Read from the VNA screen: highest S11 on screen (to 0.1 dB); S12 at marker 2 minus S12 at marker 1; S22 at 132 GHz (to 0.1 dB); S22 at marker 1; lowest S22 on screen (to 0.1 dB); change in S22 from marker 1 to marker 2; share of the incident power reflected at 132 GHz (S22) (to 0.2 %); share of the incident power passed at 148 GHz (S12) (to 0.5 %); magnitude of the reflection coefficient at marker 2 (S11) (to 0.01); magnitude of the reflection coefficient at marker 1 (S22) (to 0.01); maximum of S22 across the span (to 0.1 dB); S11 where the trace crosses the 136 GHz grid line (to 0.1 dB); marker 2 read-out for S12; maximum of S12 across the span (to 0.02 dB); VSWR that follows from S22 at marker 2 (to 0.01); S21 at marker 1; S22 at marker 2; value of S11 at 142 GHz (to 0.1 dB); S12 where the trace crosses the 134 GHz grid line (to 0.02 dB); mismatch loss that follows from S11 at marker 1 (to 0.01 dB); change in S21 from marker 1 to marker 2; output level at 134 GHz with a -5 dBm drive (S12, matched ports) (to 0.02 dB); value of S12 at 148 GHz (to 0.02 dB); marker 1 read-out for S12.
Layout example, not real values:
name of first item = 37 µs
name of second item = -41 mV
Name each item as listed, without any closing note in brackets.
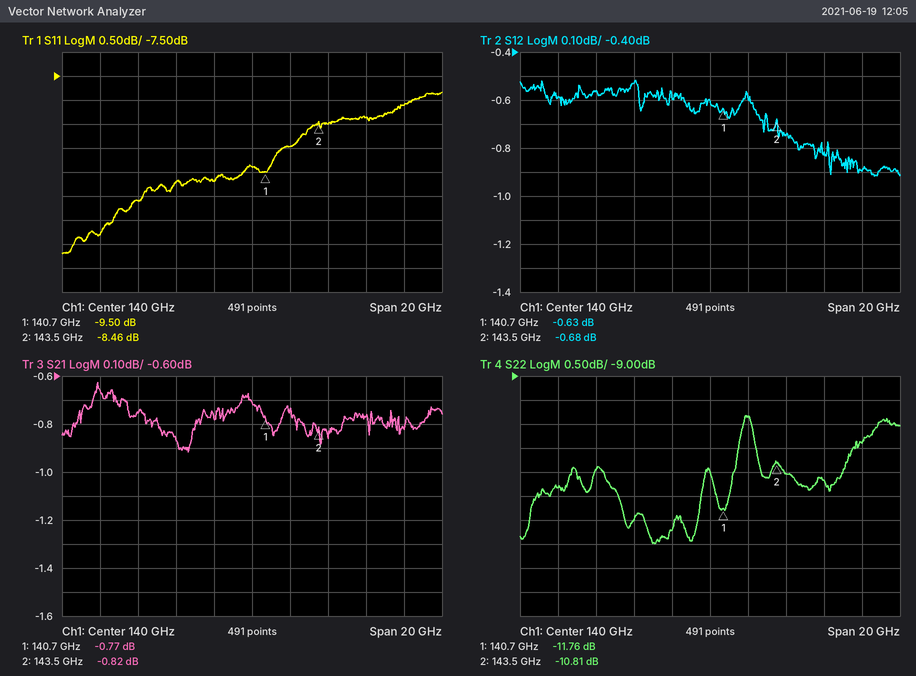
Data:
highest S11 on screen = -7.8 dB
S12 at marker 2 minus S12 at marker 1 = -0.05 dB
S22 at 132 GHz = -11.3 dB
S22 at marker 1 = -11.76 dB
lowest S22 on screen = -12.5 dB
change in S22 from marker 1 to marker 2 = 0.95 dB
share of the incident power reflected at 132 GHz (S22) = 7.4 %
share of the incident power passed at 148 GHz (S12) = 81.5 %
magnitude of the reflection coefficient at marker 2 (S11) = 0.38
magnitude of the reflection coefficient at marker 1 (S22) = 0.26
maximum of S22 across the span = -9.8 dB
S11 where the trace crosses the 136 GHz grid line = -9.7 dB
marker 2 read-out for S12 = -0.68 dB
maximum of S12 across the span = -0.52 dB
VSWR that follows from S22 at marker 2 = 1.81
S21 at marker 1 = -0.77 dB
S22 at marker 2 = -10.81 dB
value of S11 at 142 GHz = -9.0 dB
S12 where the trace crosses the 134 GHz grid line = -0.56 dB
mismatch loss that follows from S11 at marker 1 = 0.52 dB
change in S21 from marker 1 to marker 2 = -0.05 dB
output level at 134 GHz with a -5 dBm drive (S12, matched ports) = -5.56 dBm
value of S12 at 148 GHz = -0.90 dB
marker 1 read-out for S12 = -0.63 dB
